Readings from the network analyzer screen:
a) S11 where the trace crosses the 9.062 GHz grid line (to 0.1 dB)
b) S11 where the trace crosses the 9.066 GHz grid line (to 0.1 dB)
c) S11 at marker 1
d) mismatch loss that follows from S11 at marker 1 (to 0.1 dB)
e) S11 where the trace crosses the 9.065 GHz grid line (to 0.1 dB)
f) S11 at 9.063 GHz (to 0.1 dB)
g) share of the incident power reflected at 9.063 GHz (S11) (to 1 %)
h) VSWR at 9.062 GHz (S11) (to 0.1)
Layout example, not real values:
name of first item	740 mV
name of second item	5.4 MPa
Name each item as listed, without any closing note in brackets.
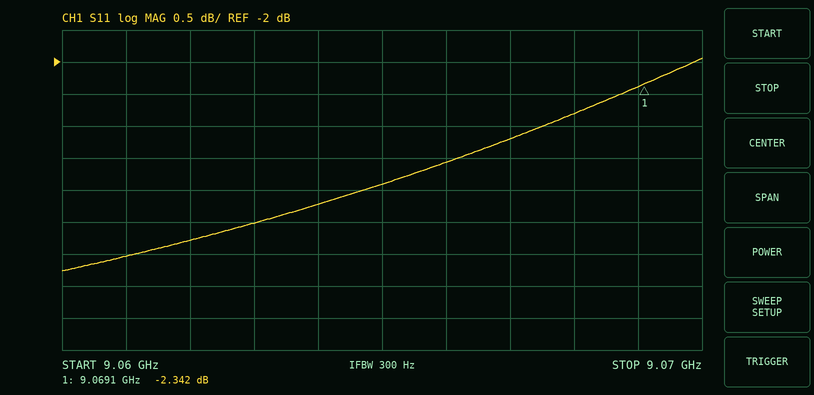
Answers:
S11 where the trace crosses the 9.062 GHz grid line	-4.8 dB
S11 where the trace crosses the 9.066 GHz grid line	-3.6 dB
S11 at marker 1	-2.342 dB
mismatch loss that follows from S11 at marker 1	3.8 dB
S11 where the trace crosses the 9.065 GHz grid line	-3.9 dB
S11 at 9.063 GHz	-4.5 dB
share of the incident power reflected at 9.063 GHz (S11)	35 %
VSWR at 9.062 GHz (S11)	3.7
